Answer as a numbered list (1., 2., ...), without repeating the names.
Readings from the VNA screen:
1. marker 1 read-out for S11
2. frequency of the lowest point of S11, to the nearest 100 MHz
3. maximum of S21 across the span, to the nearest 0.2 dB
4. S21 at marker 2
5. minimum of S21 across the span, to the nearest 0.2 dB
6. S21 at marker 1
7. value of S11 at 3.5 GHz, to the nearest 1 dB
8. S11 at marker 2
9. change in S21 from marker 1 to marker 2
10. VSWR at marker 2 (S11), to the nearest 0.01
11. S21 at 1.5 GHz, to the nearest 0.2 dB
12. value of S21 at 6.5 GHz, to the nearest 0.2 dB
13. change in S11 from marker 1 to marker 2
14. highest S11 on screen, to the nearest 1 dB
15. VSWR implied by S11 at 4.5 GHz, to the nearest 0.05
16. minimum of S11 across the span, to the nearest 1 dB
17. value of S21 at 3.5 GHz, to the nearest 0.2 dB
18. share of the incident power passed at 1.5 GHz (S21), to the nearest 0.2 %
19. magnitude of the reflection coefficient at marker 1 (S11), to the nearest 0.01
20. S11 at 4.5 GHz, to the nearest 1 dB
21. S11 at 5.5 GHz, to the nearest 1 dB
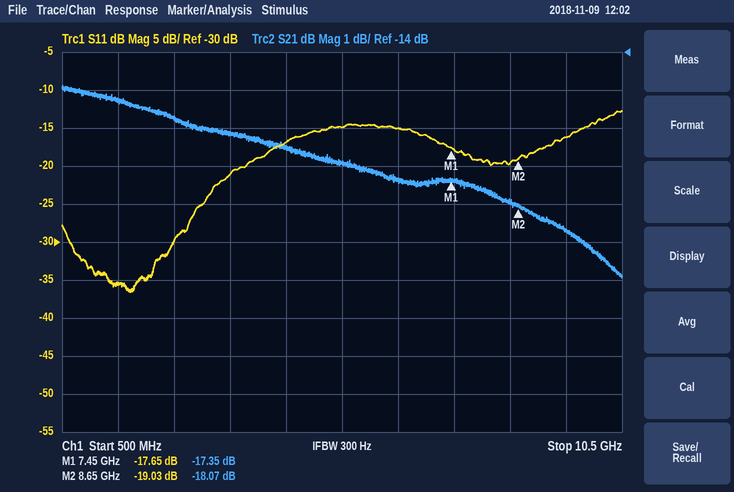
1. -17.65 dB
2. 1.7 GHz
3. -14.8 dB
4. -18.07 dB
5. -20.0 dB
6. -17.35 dB
7. -21 dB
8. -19.03 dB
9. -0.72 dB
10. 1.25
11. -15.2 dB
12. -17.4 dB
13. -1.38 dB
14. -13 dB
15. 1.35
16. -37 dB
17. -16.2 dB
18. 3.0 %
19. 0.13
20. -17 dB
21. -15 dB
